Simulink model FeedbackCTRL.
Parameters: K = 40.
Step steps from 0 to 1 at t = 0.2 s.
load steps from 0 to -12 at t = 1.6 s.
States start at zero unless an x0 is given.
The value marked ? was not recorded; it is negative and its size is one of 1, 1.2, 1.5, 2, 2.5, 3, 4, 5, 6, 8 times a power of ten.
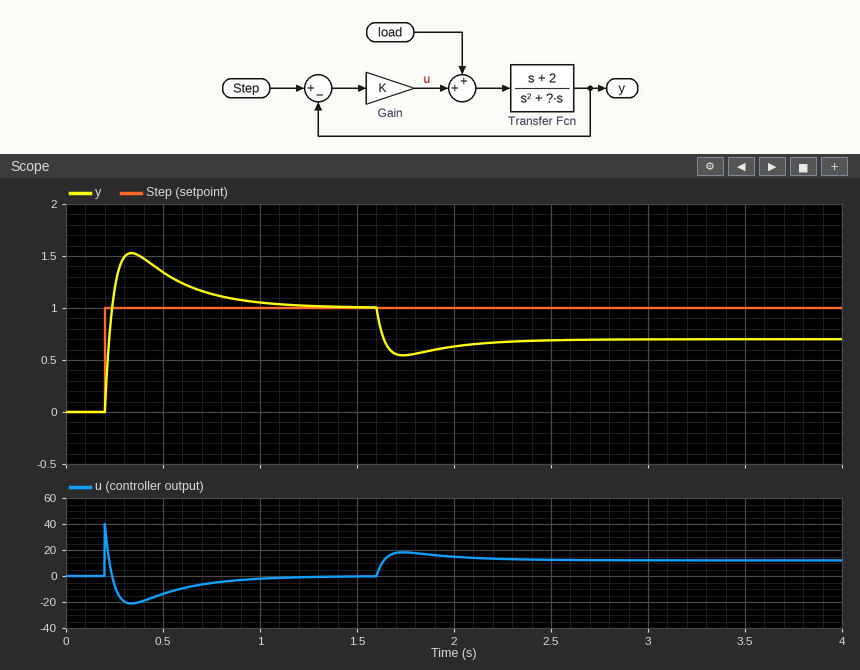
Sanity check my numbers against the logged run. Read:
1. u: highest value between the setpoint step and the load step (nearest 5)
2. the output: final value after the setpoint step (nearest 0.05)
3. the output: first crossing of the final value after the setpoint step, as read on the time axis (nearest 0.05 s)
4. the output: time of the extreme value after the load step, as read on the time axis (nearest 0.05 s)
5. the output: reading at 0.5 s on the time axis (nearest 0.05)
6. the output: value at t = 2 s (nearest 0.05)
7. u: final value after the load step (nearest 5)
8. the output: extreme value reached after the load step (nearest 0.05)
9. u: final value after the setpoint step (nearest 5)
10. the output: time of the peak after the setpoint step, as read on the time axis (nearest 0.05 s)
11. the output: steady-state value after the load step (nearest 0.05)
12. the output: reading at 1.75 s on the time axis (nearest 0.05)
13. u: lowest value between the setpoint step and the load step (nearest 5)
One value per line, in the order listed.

40
1.00
0.25 s
1.75 s
1.35
0.65
10
0.55
0
0.35 s
0.70
0.55
-20
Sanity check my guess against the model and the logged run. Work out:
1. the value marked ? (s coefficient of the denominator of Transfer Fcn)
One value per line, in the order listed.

-15
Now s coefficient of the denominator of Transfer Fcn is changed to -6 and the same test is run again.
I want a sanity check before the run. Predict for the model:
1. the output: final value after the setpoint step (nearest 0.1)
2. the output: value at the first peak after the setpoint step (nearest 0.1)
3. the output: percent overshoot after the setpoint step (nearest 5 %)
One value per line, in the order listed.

1.0
1.2
20 %
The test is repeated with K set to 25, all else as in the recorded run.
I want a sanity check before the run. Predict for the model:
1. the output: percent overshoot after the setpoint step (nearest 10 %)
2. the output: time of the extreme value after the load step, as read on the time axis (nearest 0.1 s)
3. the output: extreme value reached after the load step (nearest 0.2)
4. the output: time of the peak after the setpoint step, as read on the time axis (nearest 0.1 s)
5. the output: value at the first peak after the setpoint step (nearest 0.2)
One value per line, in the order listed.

100 %
1.8 s
0.0
0.4 s
2.0
